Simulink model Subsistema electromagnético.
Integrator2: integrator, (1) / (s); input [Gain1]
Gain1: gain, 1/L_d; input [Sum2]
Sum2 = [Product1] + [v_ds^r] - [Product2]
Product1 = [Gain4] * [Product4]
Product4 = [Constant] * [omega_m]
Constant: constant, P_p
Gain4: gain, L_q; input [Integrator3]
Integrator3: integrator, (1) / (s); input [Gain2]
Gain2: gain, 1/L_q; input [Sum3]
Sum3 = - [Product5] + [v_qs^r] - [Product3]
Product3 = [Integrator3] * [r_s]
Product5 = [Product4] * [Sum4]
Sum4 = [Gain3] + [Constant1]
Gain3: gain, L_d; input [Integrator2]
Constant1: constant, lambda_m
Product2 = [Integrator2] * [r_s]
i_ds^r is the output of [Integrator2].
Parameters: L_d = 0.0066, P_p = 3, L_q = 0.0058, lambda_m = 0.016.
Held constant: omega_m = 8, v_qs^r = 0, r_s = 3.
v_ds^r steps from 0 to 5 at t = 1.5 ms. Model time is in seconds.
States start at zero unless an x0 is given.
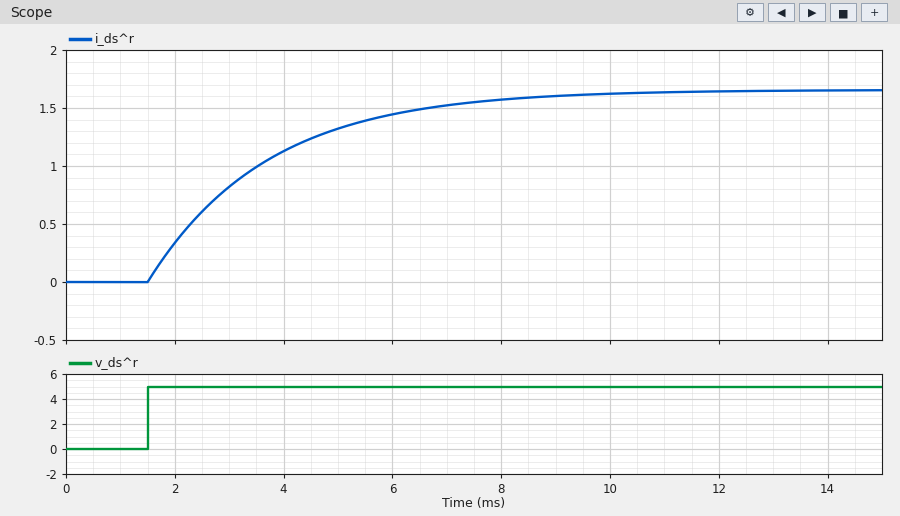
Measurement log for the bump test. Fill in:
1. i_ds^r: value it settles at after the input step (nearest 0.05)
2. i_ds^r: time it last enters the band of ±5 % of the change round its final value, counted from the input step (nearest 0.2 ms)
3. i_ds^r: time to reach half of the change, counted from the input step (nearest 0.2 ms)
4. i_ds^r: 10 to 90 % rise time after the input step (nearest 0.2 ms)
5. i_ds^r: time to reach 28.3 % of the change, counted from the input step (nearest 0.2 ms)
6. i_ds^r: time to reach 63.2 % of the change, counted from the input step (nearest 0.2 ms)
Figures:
1.65
6.6 ms
1.6 ms
4.8 ms
0.8 ms
2.2 ms
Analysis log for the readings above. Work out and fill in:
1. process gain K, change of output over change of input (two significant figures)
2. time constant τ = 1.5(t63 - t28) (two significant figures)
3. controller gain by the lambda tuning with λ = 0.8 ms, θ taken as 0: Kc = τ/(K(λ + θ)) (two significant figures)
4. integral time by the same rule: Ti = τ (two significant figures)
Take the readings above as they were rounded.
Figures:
0.33
2.1 ms
8.0
2.1 ms
